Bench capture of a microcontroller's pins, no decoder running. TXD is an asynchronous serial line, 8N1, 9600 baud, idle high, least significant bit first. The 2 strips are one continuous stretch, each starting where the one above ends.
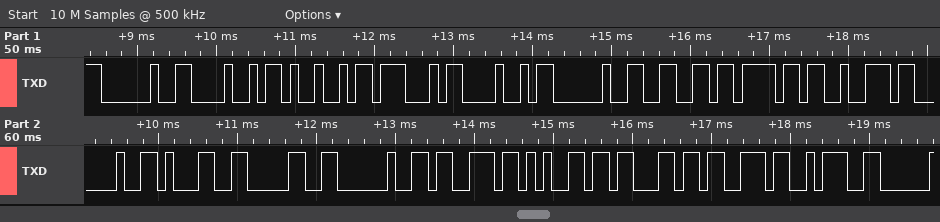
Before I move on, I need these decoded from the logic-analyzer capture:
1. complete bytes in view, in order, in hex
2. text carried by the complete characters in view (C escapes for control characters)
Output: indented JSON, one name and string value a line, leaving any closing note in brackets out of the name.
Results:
{
  "complete bytes in view, in order, in hex": "20 48 49 47 48 20 66 6F 72 20 31 30 20 73 65 63 73 3A",
  "text carried by the complete characters in view": "\" HIGH for 10 secs:\""
}
